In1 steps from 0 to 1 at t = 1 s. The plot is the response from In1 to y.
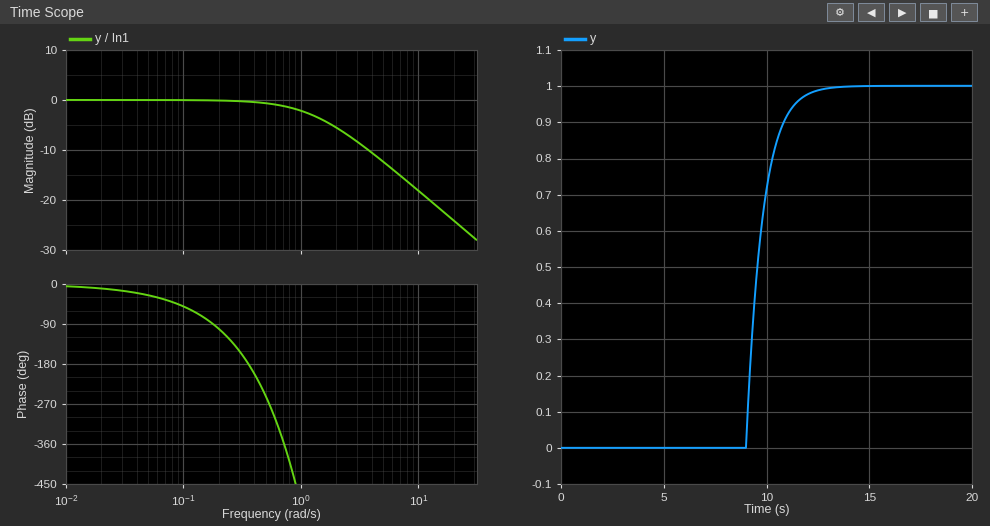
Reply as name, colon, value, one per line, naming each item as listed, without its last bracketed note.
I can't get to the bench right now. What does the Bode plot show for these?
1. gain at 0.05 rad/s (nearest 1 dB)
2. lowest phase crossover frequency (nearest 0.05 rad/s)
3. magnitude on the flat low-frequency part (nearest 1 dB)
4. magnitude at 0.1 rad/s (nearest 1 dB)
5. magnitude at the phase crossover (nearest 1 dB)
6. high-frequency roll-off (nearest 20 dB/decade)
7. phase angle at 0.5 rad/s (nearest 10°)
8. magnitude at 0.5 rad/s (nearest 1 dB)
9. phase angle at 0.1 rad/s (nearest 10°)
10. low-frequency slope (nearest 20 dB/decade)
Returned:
gain at 0.05 rad/s: 0 dB
lowest phase crossover frequency: 0.35 rad/s
magnitude on the flat low-frequency part: 0 dB
magnitude at 0.1 rad/s: 0 dB
magnitude at the phase crossover: 0 dB
high-frequency roll-off: -20 dB/decade
phase angle at 0.5 rad/s: -250°
magnitude at 0.5 rad/s: -1 dB
phase angle at 0.1 rad/s: -50°
low-frequency slope: 0 dB/decade
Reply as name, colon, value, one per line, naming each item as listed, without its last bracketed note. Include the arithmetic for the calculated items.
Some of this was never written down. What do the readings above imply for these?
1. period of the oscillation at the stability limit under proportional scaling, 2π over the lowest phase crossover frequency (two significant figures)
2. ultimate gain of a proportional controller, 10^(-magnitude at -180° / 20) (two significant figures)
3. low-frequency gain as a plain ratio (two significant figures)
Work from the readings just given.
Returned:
period of the oscillation at the stability limit under proportional scaling, 2π over the lowest phase crossover frequency: 2π / 0.35 = 18 s
ultimate gain of a proportional controller, 10^(-magnitude at -180° / 20): 10^(-0 / 20) = 1.0
low-frequency gain as a plain ratio: 10^(0 / 20) = 1.0
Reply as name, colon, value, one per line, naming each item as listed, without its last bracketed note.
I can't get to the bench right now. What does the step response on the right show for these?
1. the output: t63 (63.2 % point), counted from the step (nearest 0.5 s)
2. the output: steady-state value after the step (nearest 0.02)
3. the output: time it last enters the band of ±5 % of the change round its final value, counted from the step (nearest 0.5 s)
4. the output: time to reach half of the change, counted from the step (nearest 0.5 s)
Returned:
the output: t63 (63.2 % point), counted from the step: 9.0 s
the output: steady-state value after the step: 1.00
the output: time it last enters the band of ±5 % of the change round its final value, counted from the step: 10.5 s
the output: time to reach half of the change, counted from the step: 8.5 s
